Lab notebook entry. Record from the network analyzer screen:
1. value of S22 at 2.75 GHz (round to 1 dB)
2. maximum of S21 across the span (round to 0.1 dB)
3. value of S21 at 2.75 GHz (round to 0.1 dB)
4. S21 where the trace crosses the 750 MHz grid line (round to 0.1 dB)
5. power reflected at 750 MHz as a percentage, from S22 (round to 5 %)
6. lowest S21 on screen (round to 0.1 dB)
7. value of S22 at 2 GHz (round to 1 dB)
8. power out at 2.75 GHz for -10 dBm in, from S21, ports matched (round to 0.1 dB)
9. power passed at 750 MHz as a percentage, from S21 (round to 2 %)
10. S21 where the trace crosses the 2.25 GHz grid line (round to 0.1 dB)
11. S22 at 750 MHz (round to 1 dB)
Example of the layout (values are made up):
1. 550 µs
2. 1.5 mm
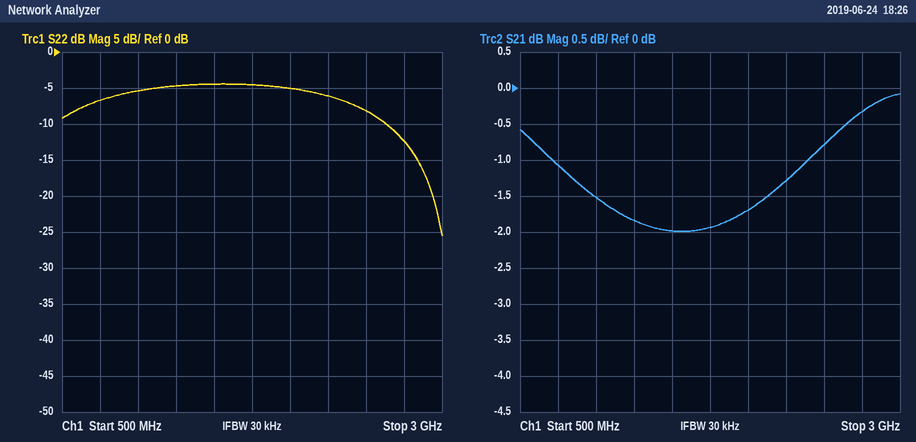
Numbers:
1. -12 dB
2. -0.1 dB
3. -0.3 dB
4. -1.1 dB
5. 20 %
6. -2.0 dB
7. -5 dB
8. -10.3 dBm
9. 78 %
10. -1.3 dB
11. -7 dB
